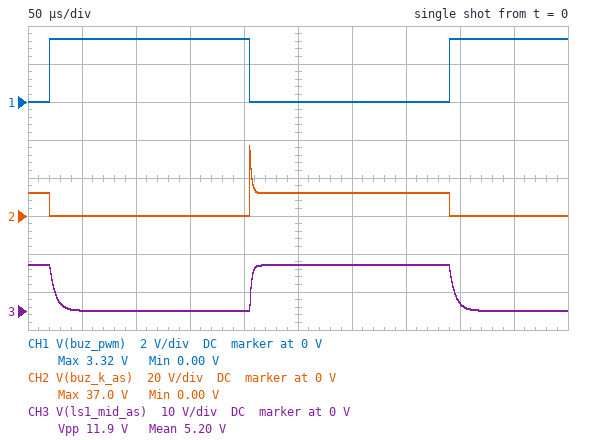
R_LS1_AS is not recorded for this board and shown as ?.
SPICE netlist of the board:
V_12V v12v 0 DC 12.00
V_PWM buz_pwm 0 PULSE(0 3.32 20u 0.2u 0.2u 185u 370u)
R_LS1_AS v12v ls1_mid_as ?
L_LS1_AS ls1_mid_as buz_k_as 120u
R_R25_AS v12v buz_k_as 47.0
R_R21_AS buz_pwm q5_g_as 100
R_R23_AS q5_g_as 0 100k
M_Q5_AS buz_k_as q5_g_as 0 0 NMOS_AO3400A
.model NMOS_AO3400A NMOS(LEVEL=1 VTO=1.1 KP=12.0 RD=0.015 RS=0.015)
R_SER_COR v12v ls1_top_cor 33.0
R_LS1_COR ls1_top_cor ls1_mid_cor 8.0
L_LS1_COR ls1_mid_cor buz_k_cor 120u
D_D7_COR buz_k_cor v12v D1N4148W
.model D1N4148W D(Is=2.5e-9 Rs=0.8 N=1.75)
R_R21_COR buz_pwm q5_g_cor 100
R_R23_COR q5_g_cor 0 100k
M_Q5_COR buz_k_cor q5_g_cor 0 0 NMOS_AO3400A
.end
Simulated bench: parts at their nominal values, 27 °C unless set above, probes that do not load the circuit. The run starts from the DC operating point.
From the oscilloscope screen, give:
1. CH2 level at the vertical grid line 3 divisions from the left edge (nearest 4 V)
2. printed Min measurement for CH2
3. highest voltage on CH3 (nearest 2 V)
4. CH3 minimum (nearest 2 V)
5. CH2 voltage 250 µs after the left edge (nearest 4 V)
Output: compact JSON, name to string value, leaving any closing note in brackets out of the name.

{"CH2 level at the vertical grid line 3 divisions from the left edge": "0 V", "printed Min measurement for CH2": "0.00 V", "highest voltage on CH3": "12 V", "CH3 minimum": "0 V", "CH2 voltage 250 µs after the left edge": "12 V"}
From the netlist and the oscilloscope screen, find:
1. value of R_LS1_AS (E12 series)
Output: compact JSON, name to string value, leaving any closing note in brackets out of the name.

{"value of R_LS1_AS": "22 Ω"}
